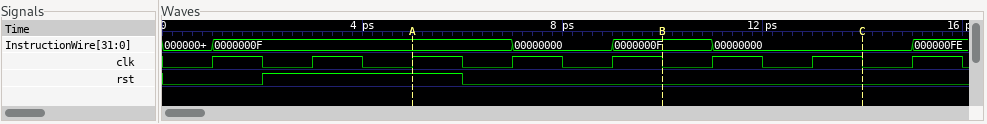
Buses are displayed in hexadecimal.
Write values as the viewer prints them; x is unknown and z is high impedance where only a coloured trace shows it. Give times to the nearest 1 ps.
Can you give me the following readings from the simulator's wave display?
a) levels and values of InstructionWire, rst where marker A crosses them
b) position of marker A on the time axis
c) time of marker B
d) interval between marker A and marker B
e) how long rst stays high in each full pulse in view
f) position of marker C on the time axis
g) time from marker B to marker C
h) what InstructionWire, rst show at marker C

InstructionWire=0000000F, rst=1
5 ps
10 ps
5 ps
4 ps
14 ps
4 ps
InstructionWire=00000000, rst=0
